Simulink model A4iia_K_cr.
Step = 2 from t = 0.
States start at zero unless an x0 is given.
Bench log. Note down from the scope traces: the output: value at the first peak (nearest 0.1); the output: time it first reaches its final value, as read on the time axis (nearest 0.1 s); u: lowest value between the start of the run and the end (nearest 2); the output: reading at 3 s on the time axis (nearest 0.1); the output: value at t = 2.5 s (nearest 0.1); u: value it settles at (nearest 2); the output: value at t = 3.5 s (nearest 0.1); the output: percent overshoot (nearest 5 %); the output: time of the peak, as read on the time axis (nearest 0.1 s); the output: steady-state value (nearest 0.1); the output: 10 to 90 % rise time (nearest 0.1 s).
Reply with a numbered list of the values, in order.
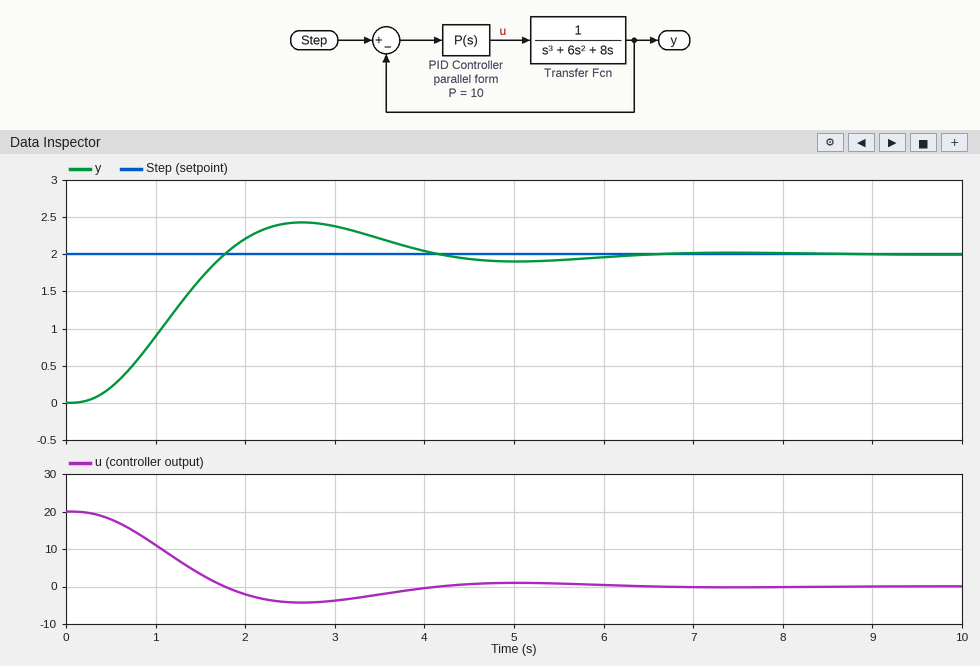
1. 2.4
2. 1.8 s
3. -4
4. 2.4
5. 2.4
6. 0
7. 2.2
8. 20 %
9. 2.6 s
10. 2.0
11. 1.1 s
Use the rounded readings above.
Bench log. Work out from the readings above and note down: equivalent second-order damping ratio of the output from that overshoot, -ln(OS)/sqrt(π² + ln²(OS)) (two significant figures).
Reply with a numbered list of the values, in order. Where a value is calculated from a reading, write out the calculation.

1. ln(0.2) = -1.609; 1.609 / sqrt(9.870 + 2.590) = 0.46
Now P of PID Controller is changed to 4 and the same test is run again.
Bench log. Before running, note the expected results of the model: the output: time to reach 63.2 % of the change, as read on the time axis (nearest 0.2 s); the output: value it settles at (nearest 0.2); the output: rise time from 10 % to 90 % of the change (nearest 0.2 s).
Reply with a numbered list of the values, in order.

1. 2.2 s
2. 2.0
3. 2.8 s
